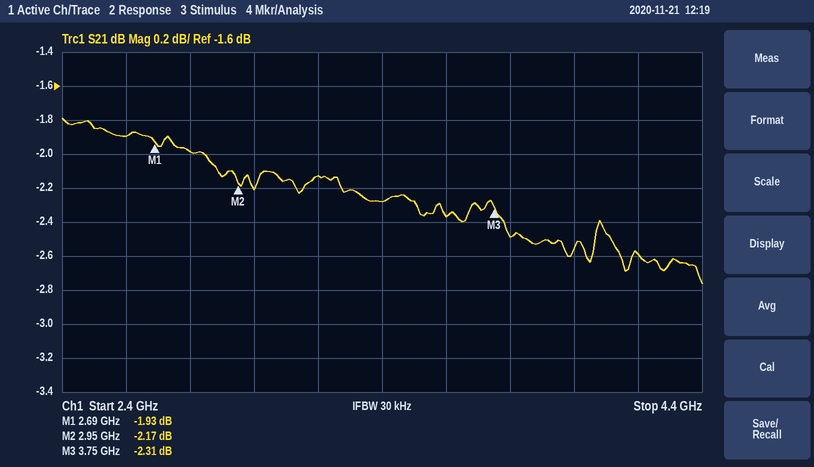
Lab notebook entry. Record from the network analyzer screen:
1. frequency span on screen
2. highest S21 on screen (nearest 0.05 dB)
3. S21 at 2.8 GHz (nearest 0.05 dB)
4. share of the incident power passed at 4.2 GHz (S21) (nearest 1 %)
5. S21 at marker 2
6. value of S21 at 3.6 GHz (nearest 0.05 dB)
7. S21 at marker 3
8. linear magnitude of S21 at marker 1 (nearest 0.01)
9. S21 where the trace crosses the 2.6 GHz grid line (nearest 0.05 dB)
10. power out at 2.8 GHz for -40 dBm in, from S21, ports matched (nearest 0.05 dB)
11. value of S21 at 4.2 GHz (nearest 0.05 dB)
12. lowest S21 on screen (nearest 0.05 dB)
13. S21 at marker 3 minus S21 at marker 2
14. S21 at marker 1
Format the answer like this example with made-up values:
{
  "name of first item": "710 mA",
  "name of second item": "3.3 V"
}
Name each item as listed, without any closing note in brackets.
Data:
{
  "frequency span on screen": "2 GHz",
  "highest S21 on screen": "-1.80 dB",
  "S21 at 2.8 GHz": "-2.00 dB",
  "share of the incident power passed at 4.2 GHz (S21)": "55 %",
  "S21 at marker 2": "-2.17 dB",
  "value of S21 at 3.6 GHz": "-2.35 dB",
  "S21 at marker 3": "-2.31 dB",
  "linear magnitude of S21 at marker 1": "0.80",
  "S21 where the trace crosses the 2.6 GHz grid line": "-1.90 dB",
  "power out at 2.8 GHz for -40 dBm in, from S21, ports matched": "-42.00 dBm",
  "value of S21 at 4.2 GHz": "-2.60 dB",
  "lowest S21 on screen": "-2.75 dB",
  "S21 at marker 3 minus S21 at marker 2": "-0.14 dB",
  "S21 at marker 1": "-1.93 dB"
}
